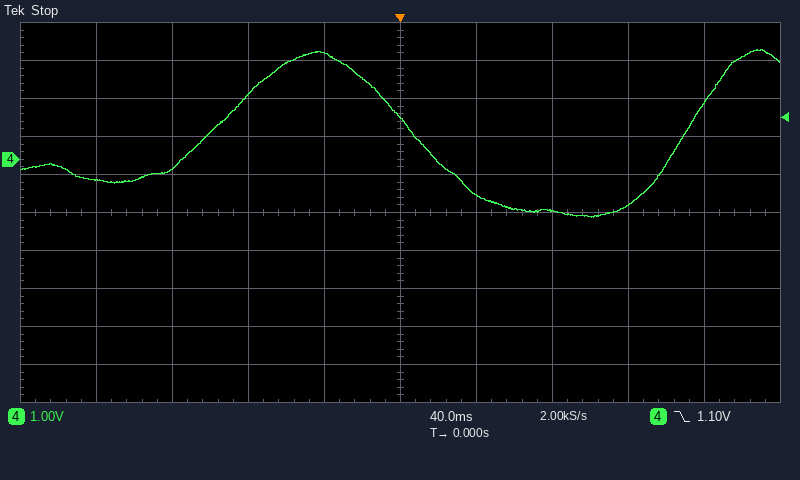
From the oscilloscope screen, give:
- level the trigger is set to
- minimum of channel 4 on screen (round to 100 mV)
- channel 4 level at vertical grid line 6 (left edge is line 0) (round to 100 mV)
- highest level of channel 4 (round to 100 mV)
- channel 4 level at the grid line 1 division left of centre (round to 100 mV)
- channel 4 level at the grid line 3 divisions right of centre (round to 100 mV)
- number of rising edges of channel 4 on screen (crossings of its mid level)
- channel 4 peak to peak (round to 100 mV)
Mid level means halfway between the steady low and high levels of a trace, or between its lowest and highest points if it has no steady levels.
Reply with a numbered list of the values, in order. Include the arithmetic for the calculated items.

1. 1.10 V
2. -1.5 V
3. -900 mV
4. 2.9 V
5. 2.8 V
6. -1.2 V
7. 2
8. 2.9 V − (-1.5 V) = 4.4 V
